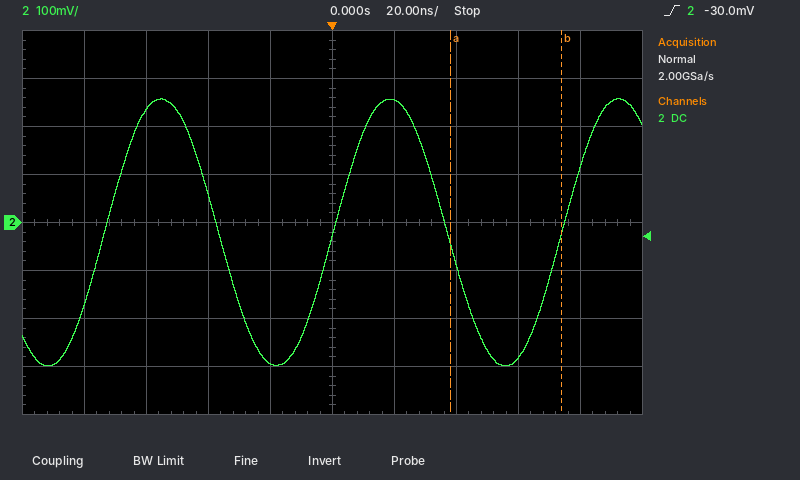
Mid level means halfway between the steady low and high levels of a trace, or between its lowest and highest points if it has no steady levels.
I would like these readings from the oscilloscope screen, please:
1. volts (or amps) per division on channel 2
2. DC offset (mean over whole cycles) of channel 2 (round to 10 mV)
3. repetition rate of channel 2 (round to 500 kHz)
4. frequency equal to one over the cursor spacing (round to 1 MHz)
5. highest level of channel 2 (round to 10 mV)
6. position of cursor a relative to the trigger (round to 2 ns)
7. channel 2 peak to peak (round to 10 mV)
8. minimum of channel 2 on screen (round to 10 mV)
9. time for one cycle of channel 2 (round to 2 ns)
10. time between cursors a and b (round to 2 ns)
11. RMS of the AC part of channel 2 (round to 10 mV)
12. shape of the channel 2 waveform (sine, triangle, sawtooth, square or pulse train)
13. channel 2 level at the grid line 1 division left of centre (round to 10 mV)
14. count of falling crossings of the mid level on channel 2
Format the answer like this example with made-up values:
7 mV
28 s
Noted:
100 mV
-20 mV
13.5 MHz
28 MHz
260 mV
+38 ns
560 mV
-300 mV
74 ns
36 ns
200 mV
sine
-290 mV
2
